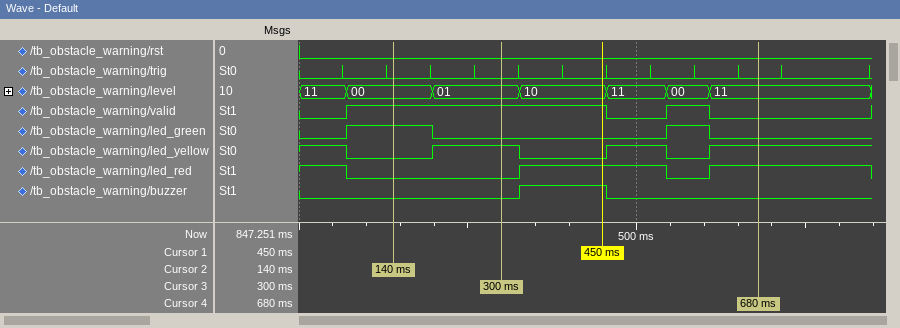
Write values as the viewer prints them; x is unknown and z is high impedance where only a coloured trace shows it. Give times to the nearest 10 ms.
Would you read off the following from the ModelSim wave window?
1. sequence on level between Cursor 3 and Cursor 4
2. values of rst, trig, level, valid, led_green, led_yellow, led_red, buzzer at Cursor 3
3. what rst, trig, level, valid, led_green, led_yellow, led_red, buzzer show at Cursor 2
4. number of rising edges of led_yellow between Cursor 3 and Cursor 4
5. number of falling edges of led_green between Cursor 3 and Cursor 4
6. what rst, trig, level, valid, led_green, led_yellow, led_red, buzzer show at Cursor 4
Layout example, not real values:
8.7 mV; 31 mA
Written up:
01, 10, 11, 00, 11; rst=0, trig=0, level=01, valid=1, led_green=0, led_yellow=1, led_red=0, buzzer=0; rst=0, trig=0, level=00, valid=1, led_green=1, led_yellow=0, led_red=0, buzzer=0; 2; 1; rst=0, trig=0, level=11, valid=0, led_green=0, led_yellow=1, led_red=1, buzzer=0
